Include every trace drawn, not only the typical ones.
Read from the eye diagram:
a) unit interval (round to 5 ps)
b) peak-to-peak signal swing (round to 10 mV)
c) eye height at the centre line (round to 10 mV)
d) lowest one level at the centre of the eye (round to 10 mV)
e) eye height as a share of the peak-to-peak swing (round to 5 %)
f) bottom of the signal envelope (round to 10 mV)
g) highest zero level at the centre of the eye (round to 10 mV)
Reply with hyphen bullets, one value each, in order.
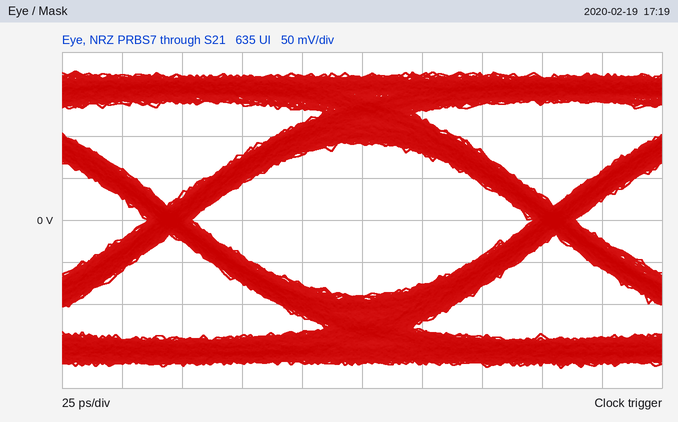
- 160 ps
- 350 mV
- 180 mV
- 90 mV
- 50 %
- -180 mV
- -90 mV
